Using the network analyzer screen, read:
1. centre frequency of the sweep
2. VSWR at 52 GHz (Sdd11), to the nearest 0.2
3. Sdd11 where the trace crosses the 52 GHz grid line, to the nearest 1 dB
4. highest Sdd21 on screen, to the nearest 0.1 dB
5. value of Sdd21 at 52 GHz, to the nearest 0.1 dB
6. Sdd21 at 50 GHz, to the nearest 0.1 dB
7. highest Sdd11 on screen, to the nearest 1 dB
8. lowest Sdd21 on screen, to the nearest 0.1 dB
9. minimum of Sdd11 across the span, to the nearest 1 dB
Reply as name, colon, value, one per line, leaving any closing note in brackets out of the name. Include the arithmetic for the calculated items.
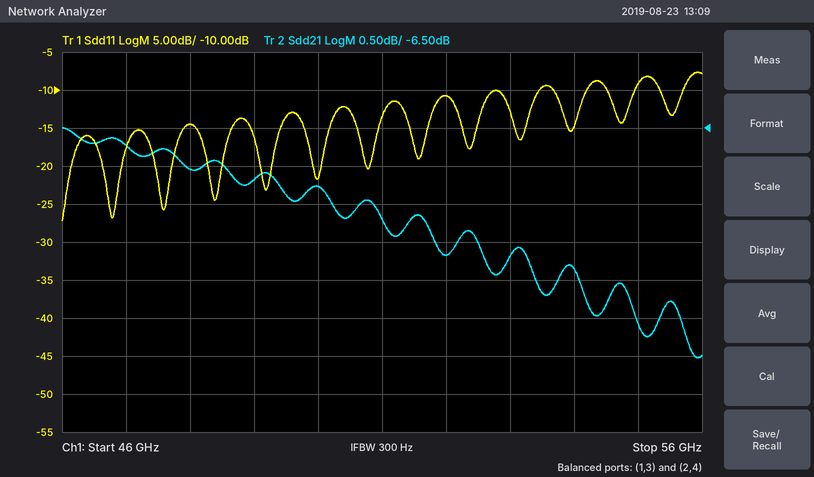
centre frequency of the sweep: 51 GHz
VSWR at 52 GHz (Sdd11), to the nearest 0.2: |Γ| = 10^(-11/20) = 0.2818; VSWR = (1 + 0.2818)/(1 − 0.2818) ≈ 1.8
Sdd11 where the trace crosses the 52 GHz grid line, to the nearest 1 dB: -11 dB
highest Sdd21 on screen, to the nearest 0.1 dB: -6.5 dB
value of Sdd21 at 52 GHz, to the nearest 0.1 dB: -8.2 dB
Sdd21 at 50 GHz, to the nearest 0.1 dB: -7.3 dB
highest Sdd11 on screen, to the nearest 1 dB: -8 dB
lowest Sdd21 on screen, to the nearest 0.1 dB: -9.5 dB
minimum of Sdd11 across the span, to the nearest 1 dB: -27 dB
